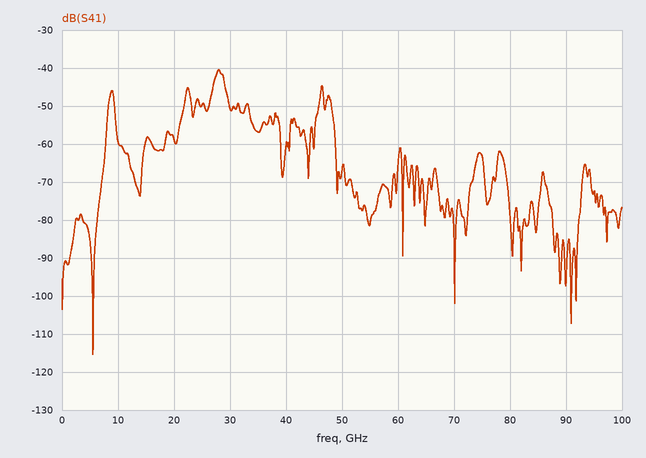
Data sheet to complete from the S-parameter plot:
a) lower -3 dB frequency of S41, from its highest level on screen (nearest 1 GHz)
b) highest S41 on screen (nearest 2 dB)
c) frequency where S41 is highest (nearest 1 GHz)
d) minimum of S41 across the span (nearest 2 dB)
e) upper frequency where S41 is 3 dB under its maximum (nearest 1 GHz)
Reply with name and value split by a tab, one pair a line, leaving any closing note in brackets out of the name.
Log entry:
lower -3 dB frequency of S41, from its highest level on screen	27 GHz
highest S41 on screen	-40 dB
frequency where S41 is highest	28 GHz
minimum of S41 across the span	-116 dB
upper frequency where S41 is 3 dB under its maximum	29 GHz
